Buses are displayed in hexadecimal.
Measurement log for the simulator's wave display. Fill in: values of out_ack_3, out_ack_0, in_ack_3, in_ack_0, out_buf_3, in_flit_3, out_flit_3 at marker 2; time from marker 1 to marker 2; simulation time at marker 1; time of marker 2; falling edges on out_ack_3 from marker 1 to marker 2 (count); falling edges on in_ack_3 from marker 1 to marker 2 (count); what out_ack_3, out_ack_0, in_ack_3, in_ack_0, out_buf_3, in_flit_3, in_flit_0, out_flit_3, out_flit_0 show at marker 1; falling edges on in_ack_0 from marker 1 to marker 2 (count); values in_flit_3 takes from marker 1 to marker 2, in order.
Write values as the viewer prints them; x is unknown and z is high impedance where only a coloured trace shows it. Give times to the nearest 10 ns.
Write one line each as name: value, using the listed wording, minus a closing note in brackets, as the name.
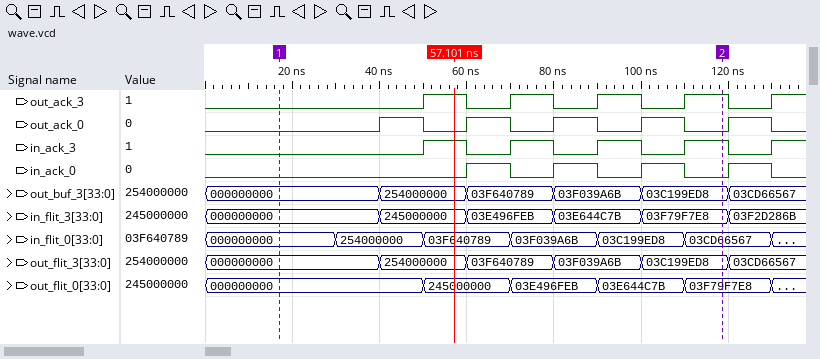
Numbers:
values of out_ack_3, out_ack_0, in_ack_3, in_ack_0, out_buf_3, in_flit_3, out_flit_3 at marker 2: out_ack_3=1, out_ack_0=0, in_ack_3=1, in_ack_0=0, out_buf_3=03C199ED8, in_flit_3=03F79F7E8, out_flit_3=03C199ED8
time from marker 1 to marker 2: 100 ns
simulation time at marker 1: 20 ns
time of marker 2: 120 ns
falling edges on out_ack_3 from marker 1 to marker 2: 3
falling edges on in_ack_3 from marker 1 to marker 2: 3
what out_ack_3, out_ack_0, in_ack_3, in_ack_0, out_buf_3, in_flit_3, in_flit_0, out_flit_3, out_flit_0 show at marker 1: out_ack_3=0, out_ack_0=0, in_ack_3=0, in_ack_0=0, out_buf_3=000000000, in_flit_3=000000000, in_flit_0=000000000, out_flit_3=000000000, out_flit_0=000000000
falling edges on in_ack_0 from marker 1 to marker 2: 3
values in_flit_3 takes from marker 1 to marker 2, in order: 000000000, 245000000, 03E496FEB, 03E644C7B, 03F79F7E8
